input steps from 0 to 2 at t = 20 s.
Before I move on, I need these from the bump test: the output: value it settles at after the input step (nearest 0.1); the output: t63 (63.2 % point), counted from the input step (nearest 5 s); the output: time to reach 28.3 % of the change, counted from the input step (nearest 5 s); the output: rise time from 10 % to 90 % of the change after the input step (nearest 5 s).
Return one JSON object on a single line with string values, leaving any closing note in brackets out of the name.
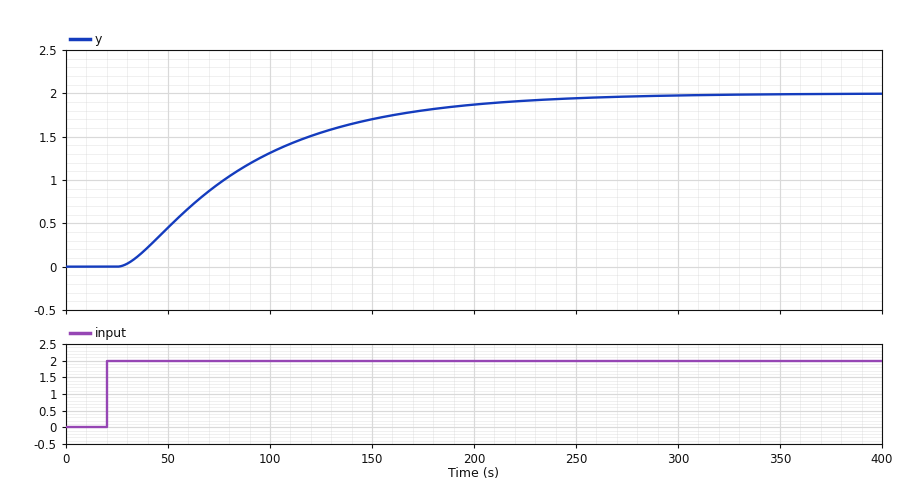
{"the output: value it settles at after the input step": "2.0", "the output: t63 (63.2 % point), counted from the input step": "75 s", "the output: time to reach 28.3 % of the change, counted from the input step": "35 s", "the output: rise time from 10 % to 90 % of the change after the input step": "135 s"}
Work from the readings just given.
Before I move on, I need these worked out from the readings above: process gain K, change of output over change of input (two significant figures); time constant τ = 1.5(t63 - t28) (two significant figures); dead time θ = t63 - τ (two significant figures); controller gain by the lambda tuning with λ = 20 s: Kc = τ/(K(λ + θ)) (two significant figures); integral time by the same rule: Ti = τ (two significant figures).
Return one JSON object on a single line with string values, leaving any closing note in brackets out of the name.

{"process gain K, change of output over change of input": "1.0", "time constant τ = 1.5(t63 - t28)": "60 s", "dead time θ = t63 - τ": "15 s", "controller gain by the lambda tuning with λ = 20 s: Kc = τ/(K(λ + θ))": "1.7", "integral time by the same rule: Ti = τ": "60 s"}
